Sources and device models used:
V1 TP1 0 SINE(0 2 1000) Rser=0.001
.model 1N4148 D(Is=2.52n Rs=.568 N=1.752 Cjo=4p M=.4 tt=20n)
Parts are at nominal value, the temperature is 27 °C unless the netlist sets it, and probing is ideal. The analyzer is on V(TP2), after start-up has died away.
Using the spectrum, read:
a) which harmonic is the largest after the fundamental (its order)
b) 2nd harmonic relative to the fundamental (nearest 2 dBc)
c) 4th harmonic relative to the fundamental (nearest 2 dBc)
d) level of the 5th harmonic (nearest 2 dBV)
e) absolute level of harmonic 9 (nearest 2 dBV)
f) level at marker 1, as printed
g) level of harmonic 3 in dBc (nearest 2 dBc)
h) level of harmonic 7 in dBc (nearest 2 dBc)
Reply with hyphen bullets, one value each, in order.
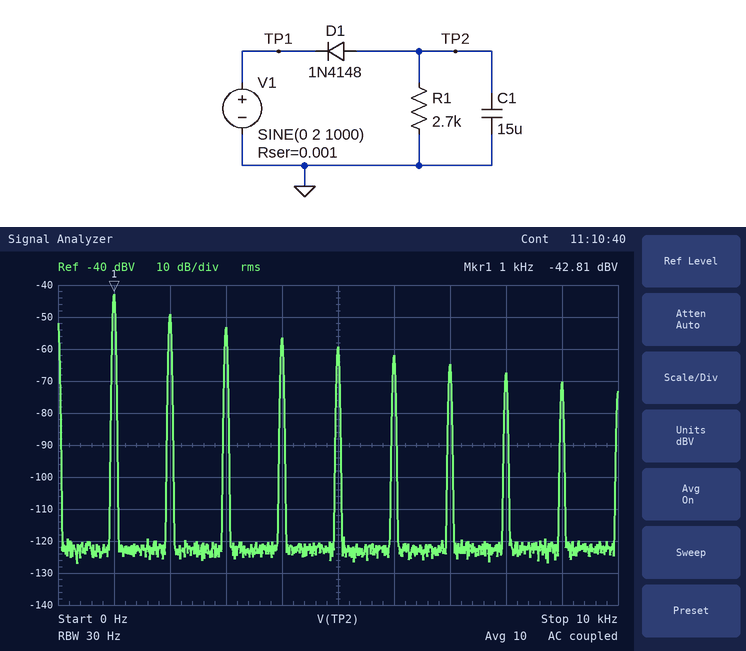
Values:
- 2
- -6 dBc
- -14 dBc
- -60 dBV
- -70 dBV
- -42.81 dBV
- -10 dBc
- -22 dBc
